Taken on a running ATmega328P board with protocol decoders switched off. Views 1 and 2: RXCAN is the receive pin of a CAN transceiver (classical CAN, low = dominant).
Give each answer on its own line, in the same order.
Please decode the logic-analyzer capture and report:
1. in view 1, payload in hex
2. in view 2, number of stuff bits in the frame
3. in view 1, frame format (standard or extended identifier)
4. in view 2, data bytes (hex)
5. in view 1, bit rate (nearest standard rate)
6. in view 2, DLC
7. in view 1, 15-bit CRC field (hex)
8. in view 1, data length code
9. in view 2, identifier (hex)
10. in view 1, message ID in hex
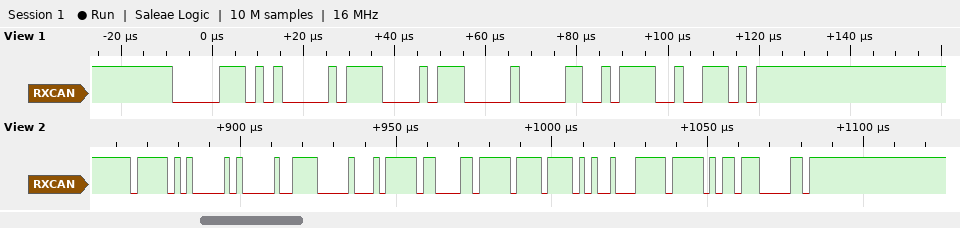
C2 E0 04
9
standard
0F 00 BF 86 FF BD 48 FF
500 kbit/s
8
0x5E4E
3
0x7E8
0x06A
